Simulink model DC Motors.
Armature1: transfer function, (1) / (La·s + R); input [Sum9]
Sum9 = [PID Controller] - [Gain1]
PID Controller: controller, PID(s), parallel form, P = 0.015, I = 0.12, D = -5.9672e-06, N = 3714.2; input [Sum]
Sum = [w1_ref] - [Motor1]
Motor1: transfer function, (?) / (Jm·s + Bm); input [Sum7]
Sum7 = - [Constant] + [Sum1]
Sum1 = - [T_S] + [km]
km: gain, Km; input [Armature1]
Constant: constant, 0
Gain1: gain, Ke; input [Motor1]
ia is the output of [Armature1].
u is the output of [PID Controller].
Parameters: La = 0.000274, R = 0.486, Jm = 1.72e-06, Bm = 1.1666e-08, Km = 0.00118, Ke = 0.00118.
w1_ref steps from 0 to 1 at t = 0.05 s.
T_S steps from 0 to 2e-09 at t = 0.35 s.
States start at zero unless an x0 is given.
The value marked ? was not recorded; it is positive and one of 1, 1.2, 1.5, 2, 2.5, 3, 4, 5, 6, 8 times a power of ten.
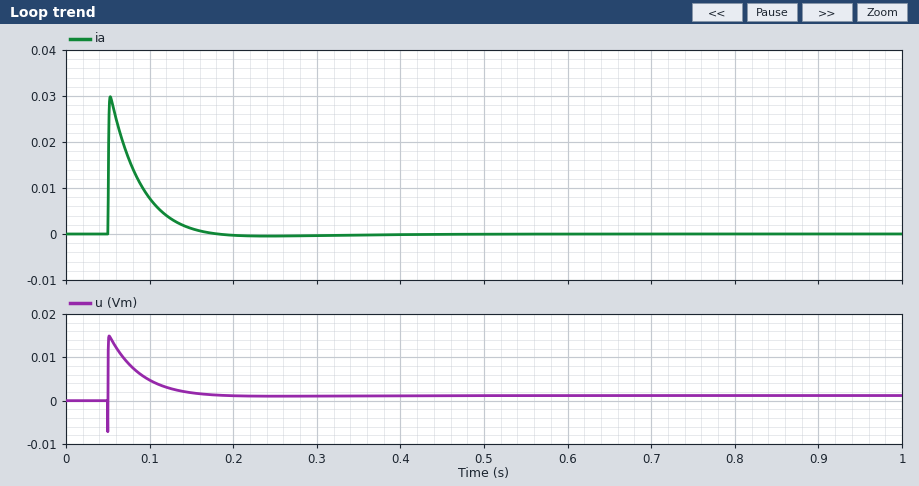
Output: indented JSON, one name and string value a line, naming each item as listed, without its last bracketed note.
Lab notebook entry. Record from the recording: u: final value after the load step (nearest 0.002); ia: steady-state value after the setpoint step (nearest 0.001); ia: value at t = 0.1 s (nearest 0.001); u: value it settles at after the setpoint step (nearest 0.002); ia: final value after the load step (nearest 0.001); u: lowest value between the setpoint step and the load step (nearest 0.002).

{
  "u: final value after the load step": "0.002",
  "ia: steady-state value after the setpoint step": "0.000",
  "ia: value at t = 0.1 s": "0.008",
  "u: value it settles at after the setpoint step": "0.002",
  "ia: final value after the load step": "0.000",
  "u: lowest value between the setpoint step and the load step": "-0.008"
}
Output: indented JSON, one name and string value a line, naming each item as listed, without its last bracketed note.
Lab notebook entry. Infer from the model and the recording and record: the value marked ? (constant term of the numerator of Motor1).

{
  "the value marked ?": "1.5"
}
